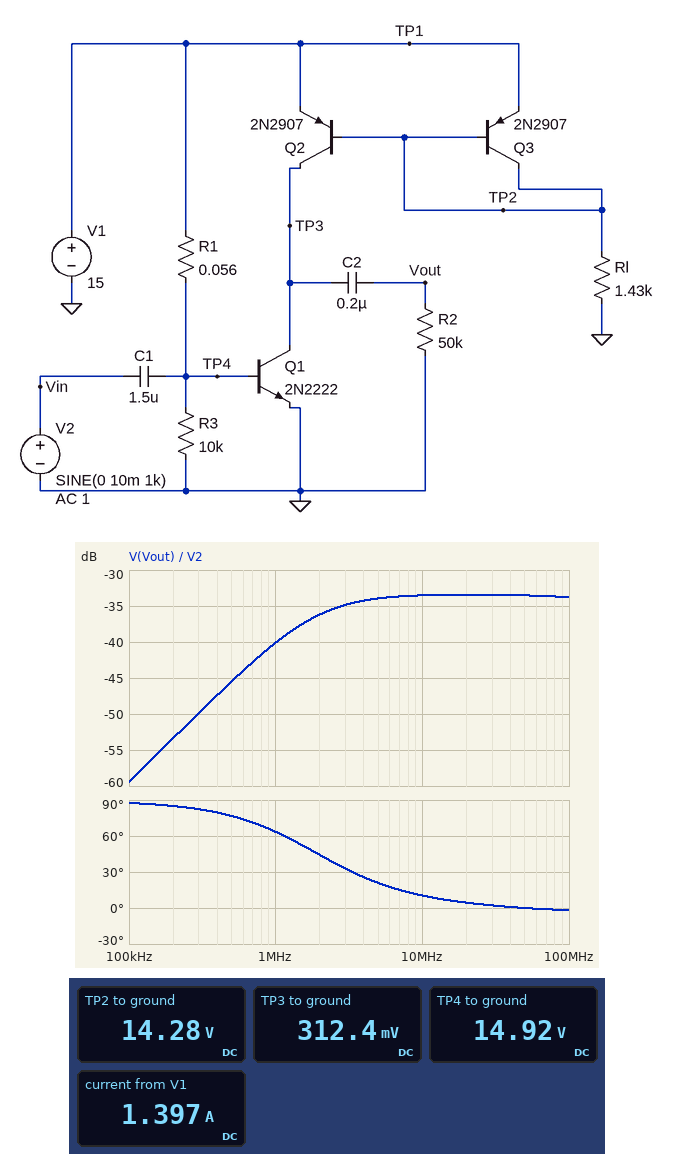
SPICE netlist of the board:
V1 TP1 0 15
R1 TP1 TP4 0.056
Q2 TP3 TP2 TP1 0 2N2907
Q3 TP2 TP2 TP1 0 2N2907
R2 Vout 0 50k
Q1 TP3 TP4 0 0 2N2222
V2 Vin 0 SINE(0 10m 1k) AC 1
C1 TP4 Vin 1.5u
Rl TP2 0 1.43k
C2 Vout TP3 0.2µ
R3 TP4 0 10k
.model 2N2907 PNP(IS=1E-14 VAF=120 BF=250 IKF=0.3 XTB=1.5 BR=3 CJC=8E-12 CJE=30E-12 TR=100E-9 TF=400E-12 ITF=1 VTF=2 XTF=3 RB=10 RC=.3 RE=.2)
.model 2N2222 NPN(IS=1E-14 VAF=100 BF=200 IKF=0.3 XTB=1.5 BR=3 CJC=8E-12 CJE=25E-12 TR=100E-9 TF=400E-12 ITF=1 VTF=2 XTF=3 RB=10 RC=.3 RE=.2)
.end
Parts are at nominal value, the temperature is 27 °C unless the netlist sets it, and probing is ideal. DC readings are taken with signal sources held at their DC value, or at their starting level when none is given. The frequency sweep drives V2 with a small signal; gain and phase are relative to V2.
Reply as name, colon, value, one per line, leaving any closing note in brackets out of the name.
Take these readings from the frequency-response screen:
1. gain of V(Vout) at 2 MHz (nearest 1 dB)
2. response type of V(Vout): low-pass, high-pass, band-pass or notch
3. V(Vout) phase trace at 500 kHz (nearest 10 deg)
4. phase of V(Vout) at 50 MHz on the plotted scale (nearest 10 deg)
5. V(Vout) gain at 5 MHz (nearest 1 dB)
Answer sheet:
gain of V(Vout) at 2 MHz: -36 dB
response type of V(Vout): low-pass, high-pass, band-pass or notch: high-pass
V(Vout) phase trace at 500 kHz: 80 deg
phase of V(Vout) at 50 MHz on the plotted scale: 0 deg
V(Vout) gain at 5 MHz: -34 dB
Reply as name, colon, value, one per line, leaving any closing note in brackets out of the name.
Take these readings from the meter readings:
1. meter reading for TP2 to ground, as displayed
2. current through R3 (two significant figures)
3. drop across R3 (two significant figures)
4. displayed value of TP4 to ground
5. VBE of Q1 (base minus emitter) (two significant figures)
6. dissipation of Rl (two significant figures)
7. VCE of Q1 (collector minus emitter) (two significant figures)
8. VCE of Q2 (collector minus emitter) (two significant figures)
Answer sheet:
meter reading for TP2 to ground, as displayed: 14.28 V
current through R3: 1.5 mA
drop across R3: 15 V
displayed value of TP4 to ground: 14.92 V
VBE of Q1 (base minus emitter): 15 V
dissipation of Rl: 140 mW
VCE of Q1 (collector minus emitter): 310 mV
VCE of Q2 (collector minus emitter): -15 V
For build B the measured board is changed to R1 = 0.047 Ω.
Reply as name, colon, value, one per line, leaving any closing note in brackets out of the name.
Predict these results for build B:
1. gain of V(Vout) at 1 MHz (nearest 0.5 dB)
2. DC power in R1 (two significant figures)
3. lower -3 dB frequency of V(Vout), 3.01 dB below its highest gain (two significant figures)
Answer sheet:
gain of V(Vout) at 1 MHz: -41.5 dB
DC power in R1: 89 mW
lower -3 dB frequency of V(Vout), 3.01 dB below its highest gain: 2.2 MHz
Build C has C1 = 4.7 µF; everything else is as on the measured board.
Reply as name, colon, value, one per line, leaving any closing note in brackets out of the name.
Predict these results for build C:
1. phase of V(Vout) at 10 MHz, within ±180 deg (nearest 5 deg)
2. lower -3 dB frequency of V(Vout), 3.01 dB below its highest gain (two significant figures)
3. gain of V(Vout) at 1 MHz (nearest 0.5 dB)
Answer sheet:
phase of V(Vout) at 10 MHz, within ±180 deg: 5 deg
lower -3 dB frequency of V(Vout), 3.01 dB below its highest gain: 630 kHz
gain of V(Vout) at 1 MHz: -35.0 dB
